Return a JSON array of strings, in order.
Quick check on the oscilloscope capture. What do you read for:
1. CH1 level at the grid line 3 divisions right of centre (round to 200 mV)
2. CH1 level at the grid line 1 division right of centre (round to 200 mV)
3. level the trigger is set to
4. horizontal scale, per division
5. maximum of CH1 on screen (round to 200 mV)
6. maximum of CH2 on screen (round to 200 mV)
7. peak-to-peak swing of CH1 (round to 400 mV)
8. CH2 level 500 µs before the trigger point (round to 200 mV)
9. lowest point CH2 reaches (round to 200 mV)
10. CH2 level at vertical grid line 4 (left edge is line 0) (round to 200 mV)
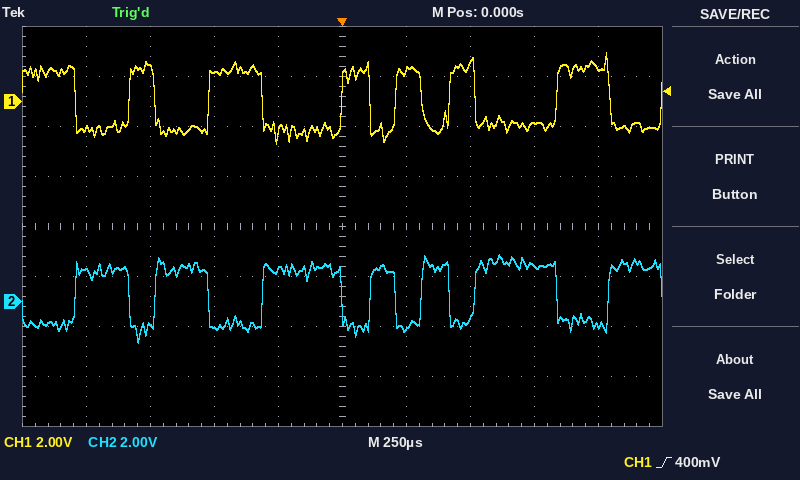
["-800 mV", "1.2 V", "400 mV", "250 µs", "2.0 V", "1.8 V", "3.6 V", "-1.0 V", "-1.6 V", "1.2 V"]
